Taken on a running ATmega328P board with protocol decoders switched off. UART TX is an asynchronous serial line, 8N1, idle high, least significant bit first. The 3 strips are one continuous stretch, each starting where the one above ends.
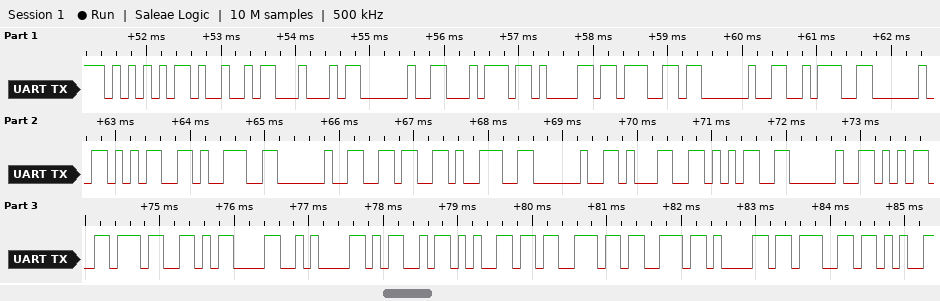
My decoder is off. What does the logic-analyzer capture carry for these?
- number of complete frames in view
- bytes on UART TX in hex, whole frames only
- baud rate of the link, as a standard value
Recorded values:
29
55 49 44 20 74 61 67 20 3A 20 35 39 20 36 39 20 31 35 20 35 37 0D 0A 4D 65 73 73 61 67
9600 baud
